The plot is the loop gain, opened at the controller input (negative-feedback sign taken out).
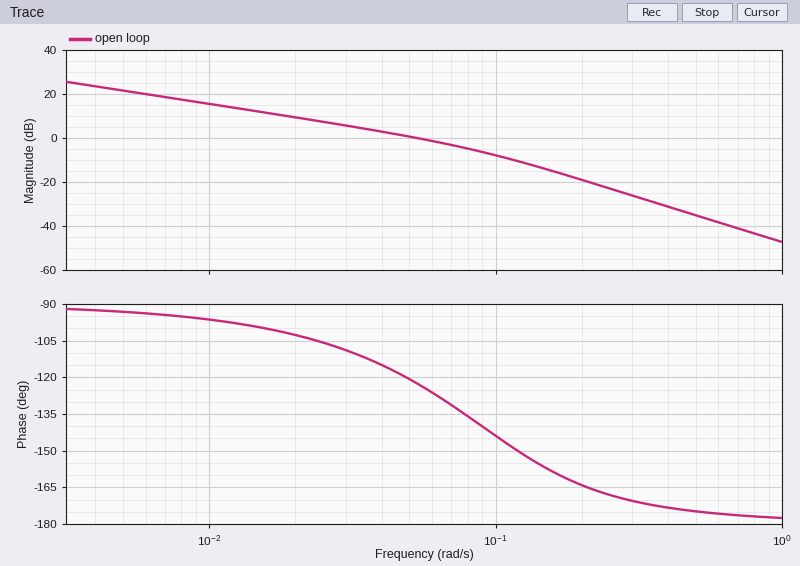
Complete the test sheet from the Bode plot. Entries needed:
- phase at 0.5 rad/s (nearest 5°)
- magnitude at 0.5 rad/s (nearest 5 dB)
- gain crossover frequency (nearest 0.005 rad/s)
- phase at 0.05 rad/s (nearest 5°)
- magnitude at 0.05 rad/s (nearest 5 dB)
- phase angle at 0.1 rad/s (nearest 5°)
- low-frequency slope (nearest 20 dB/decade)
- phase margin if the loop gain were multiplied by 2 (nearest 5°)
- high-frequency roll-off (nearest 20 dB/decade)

-175°
-35 dB
0.055 rad/s
-120°
0 dB
-145°
-20 dB/decade
40°
-40 dB/decade
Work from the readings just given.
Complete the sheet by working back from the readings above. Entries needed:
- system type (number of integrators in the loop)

1
